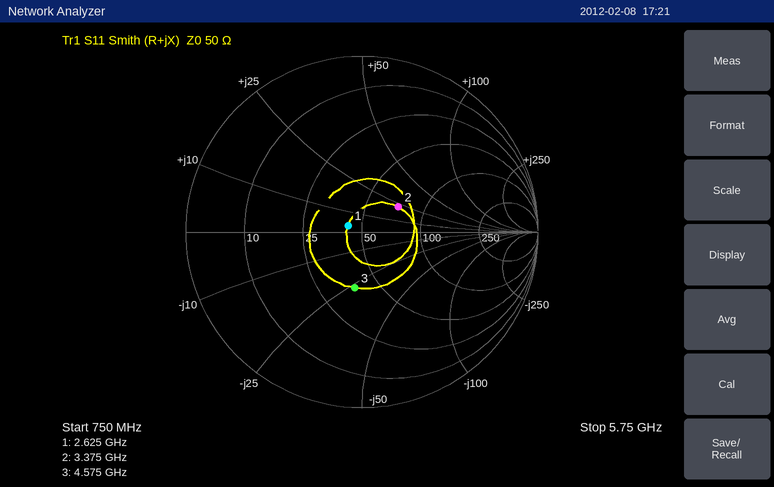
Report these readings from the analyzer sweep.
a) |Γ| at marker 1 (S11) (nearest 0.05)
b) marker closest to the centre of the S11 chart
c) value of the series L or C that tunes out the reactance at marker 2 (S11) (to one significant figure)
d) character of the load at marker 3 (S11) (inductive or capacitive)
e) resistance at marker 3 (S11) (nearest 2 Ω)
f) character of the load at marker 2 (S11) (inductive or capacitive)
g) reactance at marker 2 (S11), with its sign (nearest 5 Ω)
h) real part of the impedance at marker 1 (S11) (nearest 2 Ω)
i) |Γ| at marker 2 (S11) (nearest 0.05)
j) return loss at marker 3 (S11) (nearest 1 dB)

0.10
marker 1
2 pF
capacitive
38 Ω
inductive
+20 Ω
42 Ω
0.25
10 dB
